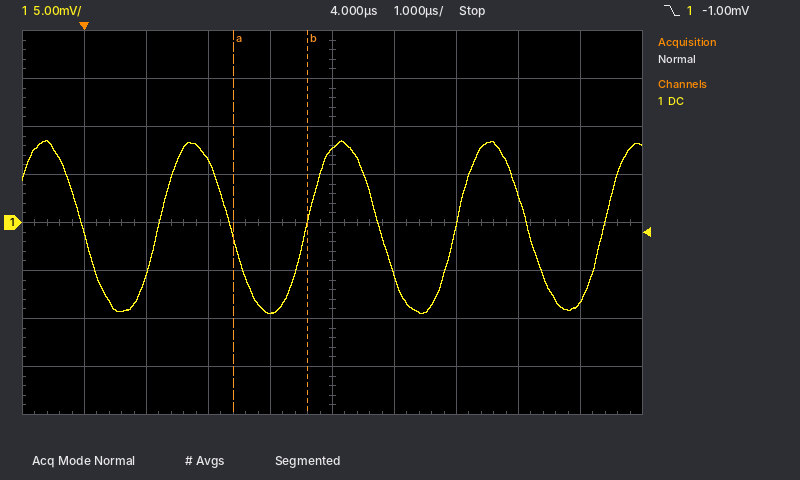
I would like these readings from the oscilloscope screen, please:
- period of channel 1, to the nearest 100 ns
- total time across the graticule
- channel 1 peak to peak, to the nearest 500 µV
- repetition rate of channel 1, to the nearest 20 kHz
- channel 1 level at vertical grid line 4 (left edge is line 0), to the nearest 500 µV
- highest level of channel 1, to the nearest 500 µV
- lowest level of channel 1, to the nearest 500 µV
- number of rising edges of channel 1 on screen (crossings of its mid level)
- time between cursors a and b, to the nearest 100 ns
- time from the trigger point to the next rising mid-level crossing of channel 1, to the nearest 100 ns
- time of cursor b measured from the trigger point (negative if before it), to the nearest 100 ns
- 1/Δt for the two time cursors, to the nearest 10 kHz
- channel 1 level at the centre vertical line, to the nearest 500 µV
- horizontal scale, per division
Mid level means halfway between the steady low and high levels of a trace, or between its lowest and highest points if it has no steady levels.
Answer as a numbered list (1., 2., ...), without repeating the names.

1. 2.4 µs
2. 10 µs
3. 18.0 mV
4. 420 kHz
5. -9.5 mV
6. 8.5 mV
7. -9.5 mV
8. 4
9. 1.2 µs
10. 1.2 µs
11. +3.6 µs
12. 830 kHz
13. 7.5 mV
14. 1 µs
